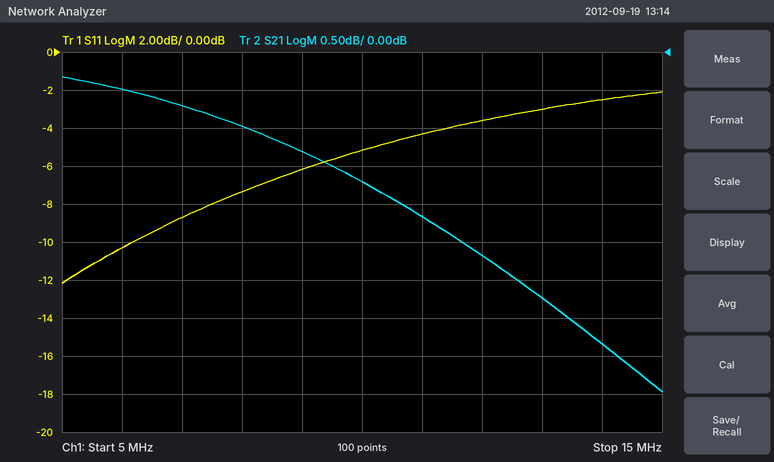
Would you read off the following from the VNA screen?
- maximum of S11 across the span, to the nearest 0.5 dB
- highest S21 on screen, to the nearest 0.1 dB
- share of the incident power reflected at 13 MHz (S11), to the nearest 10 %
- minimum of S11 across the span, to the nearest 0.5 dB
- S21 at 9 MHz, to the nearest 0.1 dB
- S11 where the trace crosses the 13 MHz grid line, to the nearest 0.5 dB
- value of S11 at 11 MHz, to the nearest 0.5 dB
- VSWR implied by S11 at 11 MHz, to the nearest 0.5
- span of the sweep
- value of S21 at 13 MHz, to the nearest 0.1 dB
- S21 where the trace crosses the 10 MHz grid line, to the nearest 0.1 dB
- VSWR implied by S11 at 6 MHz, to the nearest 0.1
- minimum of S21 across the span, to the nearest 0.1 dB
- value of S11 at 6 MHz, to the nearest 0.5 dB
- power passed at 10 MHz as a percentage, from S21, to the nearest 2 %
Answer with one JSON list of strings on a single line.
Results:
["-2.0 dB", "-0.3 dB", "50 %", "-12.0 dB", "-1.3 dB", "-3.0 dB", "-4.5 dB", "4.0", "10 MHz", "-3.2 dB", "-1.7 dB", "1.9", "-4.5 dB", "-10.5 dB", "68 %"]
